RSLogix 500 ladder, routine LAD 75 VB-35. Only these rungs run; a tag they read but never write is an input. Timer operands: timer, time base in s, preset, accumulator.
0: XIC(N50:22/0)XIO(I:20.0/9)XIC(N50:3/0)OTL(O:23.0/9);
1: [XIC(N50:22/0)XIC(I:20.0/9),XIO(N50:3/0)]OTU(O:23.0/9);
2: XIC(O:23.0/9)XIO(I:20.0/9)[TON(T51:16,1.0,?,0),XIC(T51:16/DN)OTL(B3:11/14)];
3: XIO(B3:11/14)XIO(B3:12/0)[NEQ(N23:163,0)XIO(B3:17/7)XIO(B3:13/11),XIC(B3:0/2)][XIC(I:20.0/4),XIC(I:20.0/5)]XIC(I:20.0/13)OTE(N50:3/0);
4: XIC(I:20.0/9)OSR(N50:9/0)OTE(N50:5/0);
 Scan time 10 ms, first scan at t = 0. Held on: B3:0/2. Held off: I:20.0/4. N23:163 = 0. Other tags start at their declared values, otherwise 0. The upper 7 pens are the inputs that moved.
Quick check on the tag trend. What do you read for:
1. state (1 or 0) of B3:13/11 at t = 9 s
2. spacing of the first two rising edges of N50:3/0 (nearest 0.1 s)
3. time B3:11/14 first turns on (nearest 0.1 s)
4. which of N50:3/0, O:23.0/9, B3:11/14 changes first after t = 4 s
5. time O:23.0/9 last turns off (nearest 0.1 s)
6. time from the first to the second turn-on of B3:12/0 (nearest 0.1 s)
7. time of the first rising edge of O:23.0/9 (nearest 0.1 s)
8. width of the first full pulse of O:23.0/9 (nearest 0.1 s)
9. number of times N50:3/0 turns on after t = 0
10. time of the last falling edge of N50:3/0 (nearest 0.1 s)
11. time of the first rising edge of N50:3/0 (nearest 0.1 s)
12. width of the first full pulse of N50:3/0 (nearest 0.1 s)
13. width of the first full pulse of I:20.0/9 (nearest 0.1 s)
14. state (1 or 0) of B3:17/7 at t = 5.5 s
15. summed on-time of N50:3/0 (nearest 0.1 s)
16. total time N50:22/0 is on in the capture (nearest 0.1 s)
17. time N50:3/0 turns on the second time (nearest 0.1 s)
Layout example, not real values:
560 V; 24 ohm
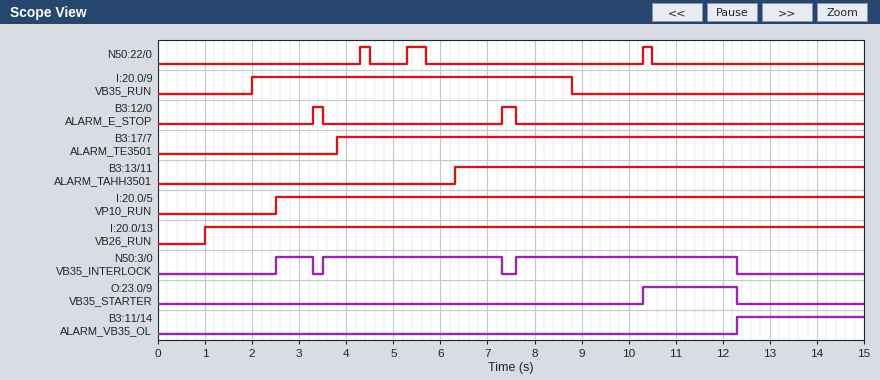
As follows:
1; 1.0 s; 12.3 s; N50:3/0; 12.3 s; 4.0 s; 10.3 s; 2.0 s; 3; 12.3 s; 2.5 s; 0.8 s; 6.8 s; 1; 9.3 s; 0.8 s; 3.5 s
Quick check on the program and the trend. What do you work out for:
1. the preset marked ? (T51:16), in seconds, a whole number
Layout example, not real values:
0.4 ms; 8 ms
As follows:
2 s
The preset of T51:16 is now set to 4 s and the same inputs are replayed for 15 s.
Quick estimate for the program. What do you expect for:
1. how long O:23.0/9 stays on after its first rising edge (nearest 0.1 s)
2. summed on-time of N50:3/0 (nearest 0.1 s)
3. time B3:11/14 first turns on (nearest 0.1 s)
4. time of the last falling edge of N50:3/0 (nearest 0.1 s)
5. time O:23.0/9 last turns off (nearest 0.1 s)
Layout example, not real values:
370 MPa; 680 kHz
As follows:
4.0 s; 11.3 s; 14.3 s; 14.3 s; 14.3 s
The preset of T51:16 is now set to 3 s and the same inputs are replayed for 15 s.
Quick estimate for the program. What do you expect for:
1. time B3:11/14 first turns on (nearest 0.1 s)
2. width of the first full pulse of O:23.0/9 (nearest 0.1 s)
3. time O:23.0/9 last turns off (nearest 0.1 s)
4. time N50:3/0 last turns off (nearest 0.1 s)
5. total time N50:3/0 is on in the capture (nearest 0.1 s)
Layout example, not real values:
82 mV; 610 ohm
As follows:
13.3 s; 3.0 s; 13.3 s; 13.3 s; 10.3 s
